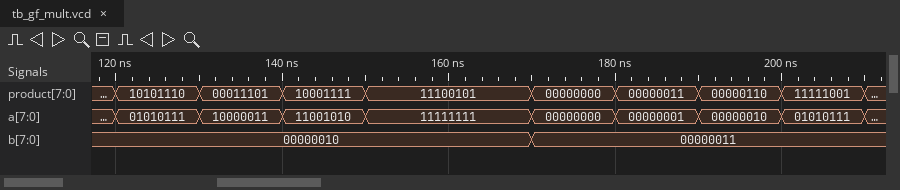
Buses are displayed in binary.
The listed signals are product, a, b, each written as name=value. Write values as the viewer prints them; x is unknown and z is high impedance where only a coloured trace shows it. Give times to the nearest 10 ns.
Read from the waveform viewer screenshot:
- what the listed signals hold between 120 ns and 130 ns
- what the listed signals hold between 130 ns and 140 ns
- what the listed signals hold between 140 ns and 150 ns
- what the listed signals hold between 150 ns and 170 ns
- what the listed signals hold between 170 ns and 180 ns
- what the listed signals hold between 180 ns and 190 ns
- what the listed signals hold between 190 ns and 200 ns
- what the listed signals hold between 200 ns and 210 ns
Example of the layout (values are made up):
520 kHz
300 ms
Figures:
product=10101110, a=01010111, b=00000010
product=00011101, a=10000011, b=00000010
product=10001111, a=11001010, b=00000010
product=11100101, a=11111111, b=00000010
product=00000000, a=00000000, b=00000011
product=00000011, a=00000001, b=00000011
product=00000110, a=00000010, b=00000011
product=11111001, a=01010111, b=00000011
